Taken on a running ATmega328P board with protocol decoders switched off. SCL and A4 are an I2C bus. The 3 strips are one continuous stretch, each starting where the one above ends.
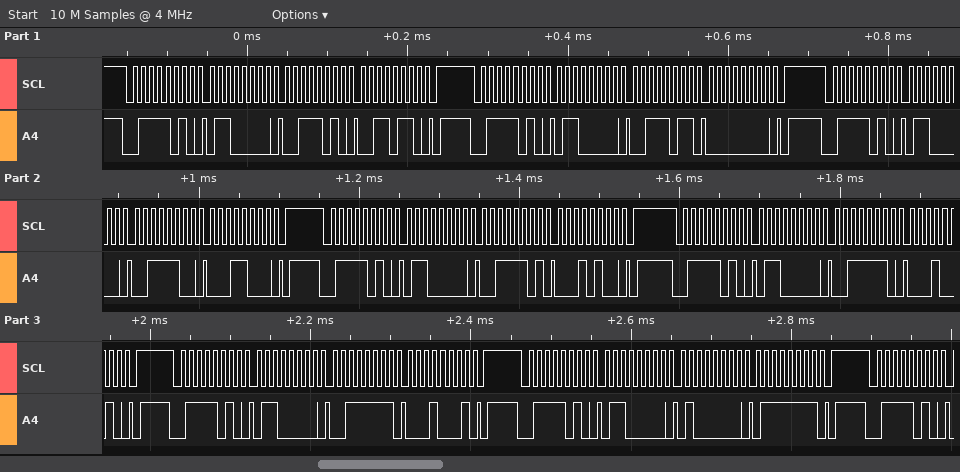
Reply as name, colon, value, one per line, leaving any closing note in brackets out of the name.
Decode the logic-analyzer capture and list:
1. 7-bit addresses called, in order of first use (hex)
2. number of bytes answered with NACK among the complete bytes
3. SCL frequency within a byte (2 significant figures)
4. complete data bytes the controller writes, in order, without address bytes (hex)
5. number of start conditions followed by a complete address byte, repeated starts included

7-bit addresses called, in order of first use: 0x3D
number of bytes answered with NACK among the complete bytes: 0
SCL frequency within a byte: 100 kHz
complete data bytes the controller writes, in order, without address bytes: 60 3A 36 60 3B 00 60 3C 18 60 3D 14 60 3E 12 60 3F 11 60 40 7F
number of start conditions followed by a complete address byte, repeated starts included: 8
